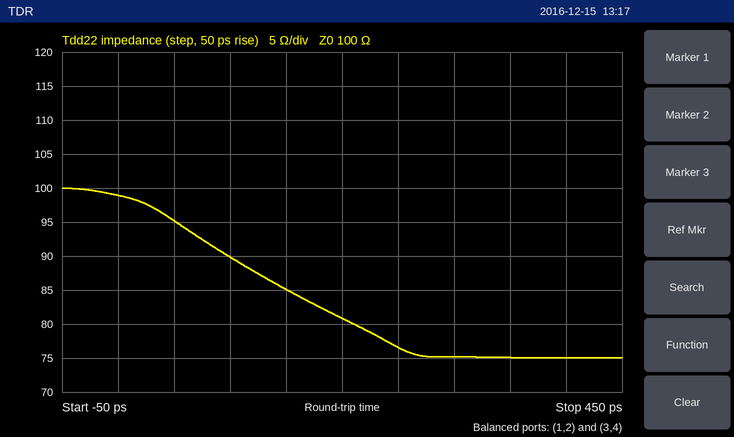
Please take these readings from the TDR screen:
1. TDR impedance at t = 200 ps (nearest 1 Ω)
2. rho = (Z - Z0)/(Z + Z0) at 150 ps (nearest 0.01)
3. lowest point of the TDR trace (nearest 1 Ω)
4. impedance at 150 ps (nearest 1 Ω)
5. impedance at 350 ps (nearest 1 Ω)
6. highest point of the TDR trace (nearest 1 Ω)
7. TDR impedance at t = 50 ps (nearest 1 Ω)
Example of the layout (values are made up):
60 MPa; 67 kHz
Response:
81 Ω; -0.08; 75 Ω; 85 Ω; 75 Ω; 100 Ω; 95 Ω
